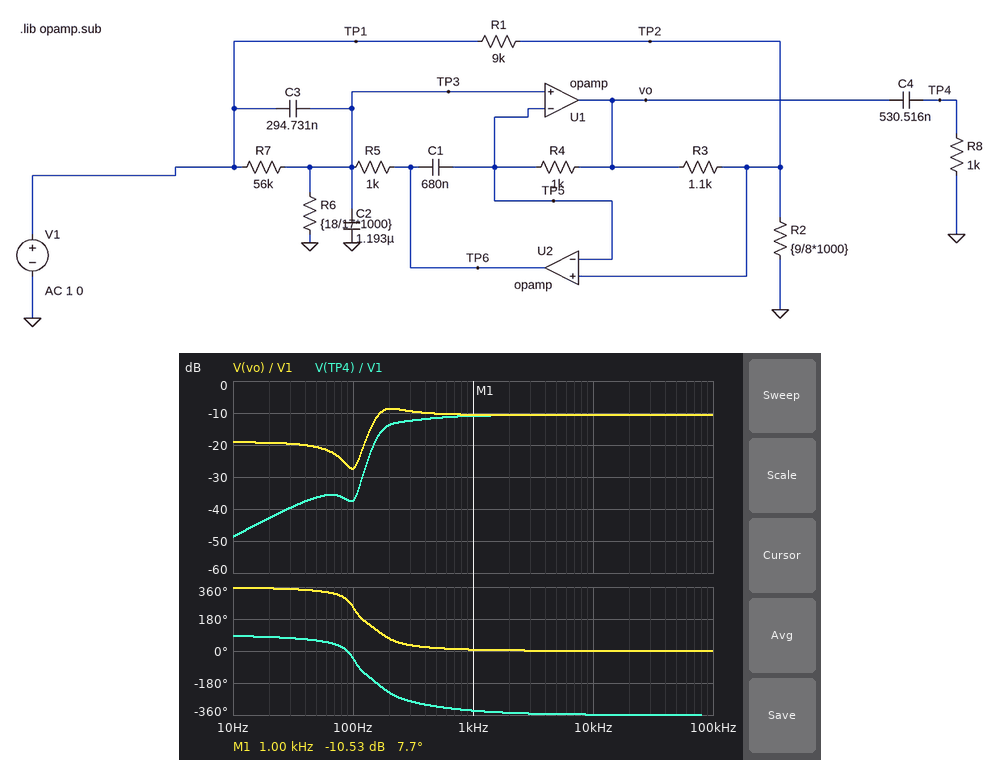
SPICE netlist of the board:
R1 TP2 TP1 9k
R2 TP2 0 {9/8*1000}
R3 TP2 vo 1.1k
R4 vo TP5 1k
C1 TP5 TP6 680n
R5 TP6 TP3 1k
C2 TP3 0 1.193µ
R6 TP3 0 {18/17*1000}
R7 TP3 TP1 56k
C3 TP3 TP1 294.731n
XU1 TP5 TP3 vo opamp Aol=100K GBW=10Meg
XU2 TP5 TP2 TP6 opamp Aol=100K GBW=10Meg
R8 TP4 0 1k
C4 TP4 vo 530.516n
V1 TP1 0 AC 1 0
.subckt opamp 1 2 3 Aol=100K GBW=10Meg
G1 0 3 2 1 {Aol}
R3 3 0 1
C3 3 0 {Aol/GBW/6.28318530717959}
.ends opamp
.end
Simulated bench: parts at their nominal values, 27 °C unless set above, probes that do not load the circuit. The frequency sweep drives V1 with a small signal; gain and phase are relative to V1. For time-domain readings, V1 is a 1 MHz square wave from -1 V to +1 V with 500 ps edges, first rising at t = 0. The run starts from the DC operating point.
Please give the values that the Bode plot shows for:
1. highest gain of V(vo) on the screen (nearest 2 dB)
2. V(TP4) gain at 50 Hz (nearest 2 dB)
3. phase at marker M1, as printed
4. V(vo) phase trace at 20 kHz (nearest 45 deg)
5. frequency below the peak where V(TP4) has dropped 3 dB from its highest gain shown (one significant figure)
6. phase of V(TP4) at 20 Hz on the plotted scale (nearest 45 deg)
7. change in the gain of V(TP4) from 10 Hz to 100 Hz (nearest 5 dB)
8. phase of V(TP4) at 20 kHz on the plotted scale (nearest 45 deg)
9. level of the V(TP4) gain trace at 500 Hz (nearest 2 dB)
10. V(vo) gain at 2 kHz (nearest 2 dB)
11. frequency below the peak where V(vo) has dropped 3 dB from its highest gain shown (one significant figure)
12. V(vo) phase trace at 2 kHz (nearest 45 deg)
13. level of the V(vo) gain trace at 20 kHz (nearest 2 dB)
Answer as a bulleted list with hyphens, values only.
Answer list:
- -8 dB
- -36 dB
- 7.7 deg
- 0 deg
- 200 Hz
- 90 deg
- 10 dB
- -360 deg
- -12 dB
- -10 dB
- 200 Hz
- 0 deg
- -10 dB
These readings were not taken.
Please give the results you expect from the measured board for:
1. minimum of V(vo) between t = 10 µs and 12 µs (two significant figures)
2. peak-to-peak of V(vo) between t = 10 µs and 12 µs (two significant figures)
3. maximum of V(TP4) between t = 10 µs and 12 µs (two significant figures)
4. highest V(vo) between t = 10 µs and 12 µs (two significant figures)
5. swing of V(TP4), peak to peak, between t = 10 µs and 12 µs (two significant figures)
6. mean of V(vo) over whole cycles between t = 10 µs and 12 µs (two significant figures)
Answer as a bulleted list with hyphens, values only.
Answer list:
- -170 mV
- 700 mV
- 630 mV
- 530 mV
- 700 mV
- 180 mV
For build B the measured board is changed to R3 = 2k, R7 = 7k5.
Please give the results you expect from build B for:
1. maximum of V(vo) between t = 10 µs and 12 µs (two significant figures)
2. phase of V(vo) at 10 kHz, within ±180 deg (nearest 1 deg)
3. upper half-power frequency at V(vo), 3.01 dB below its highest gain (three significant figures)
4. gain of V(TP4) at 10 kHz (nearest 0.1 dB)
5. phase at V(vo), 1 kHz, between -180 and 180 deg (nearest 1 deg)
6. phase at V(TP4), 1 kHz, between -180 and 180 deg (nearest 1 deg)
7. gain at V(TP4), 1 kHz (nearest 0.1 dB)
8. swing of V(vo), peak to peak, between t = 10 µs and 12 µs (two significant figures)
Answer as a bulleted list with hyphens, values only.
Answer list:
- 640 mV
- 0 deg
- 565 Hz
- -8.6 dB
- 4 deg
- 21 deg
- -8.7 dB
- 770 mV
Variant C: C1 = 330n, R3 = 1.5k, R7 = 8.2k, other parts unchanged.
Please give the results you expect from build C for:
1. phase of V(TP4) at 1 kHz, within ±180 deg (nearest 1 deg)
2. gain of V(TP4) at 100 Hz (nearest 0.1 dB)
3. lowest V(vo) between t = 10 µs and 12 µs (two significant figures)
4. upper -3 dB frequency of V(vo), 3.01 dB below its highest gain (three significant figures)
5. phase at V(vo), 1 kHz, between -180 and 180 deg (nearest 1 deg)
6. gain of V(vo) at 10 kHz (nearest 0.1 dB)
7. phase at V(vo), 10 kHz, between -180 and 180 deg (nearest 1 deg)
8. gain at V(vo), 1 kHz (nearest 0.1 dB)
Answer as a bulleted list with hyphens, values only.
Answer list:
- 21 deg
- -31.9 dB
- -150 mV
- 481 Hz
- 5 deg
- -9.7 dB
- 0 deg
- -9.3 dB
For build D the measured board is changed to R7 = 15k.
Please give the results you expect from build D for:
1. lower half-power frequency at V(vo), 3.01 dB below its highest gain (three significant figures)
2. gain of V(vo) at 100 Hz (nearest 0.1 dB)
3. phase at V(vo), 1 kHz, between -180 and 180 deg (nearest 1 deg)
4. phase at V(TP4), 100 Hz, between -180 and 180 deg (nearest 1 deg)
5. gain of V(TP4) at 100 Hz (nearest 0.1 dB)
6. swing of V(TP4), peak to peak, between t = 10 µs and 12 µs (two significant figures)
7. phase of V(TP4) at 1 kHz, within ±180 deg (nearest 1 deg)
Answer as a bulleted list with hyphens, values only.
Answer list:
- 158 Hz
- -39.7 dB
- 6 deg
- 95 deg
- -49.7 dB
- 700 mV
- 23 deg
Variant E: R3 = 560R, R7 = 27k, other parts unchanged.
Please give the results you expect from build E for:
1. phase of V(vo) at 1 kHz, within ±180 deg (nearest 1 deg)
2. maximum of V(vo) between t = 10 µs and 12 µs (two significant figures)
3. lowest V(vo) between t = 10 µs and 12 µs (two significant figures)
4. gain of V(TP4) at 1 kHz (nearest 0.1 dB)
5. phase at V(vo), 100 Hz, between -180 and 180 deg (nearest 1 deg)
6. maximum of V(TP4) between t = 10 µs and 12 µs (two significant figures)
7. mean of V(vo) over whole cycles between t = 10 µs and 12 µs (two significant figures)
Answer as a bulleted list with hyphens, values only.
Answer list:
- 6 deg
- 470 mV
- -200 mV
- -12.5 dB
- 113 deg
- 570 mV
- 130 mV
